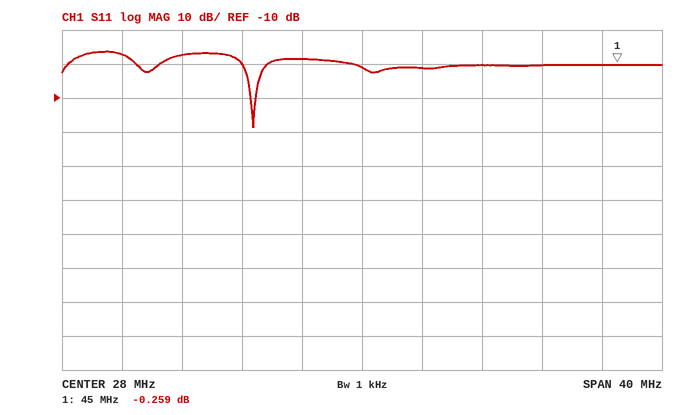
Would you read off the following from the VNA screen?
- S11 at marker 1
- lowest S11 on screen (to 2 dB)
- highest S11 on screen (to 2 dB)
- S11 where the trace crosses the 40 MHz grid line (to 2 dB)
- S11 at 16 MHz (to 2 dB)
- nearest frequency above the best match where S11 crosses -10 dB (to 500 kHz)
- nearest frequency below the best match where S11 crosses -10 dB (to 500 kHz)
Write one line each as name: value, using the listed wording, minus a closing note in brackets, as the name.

S11 at marker 1: -0.259 dB
lowest S11 on screen: -18 dB
highest S11 on screen: 4 dB
S11 where the trace crosses the 40 MHz grid line: 0 dB
S11 at 16 MHz: 2 dB
nearest frequency above the best match where S11 crosses -10 dB: 21.0 MHz
nearest frequency below the best match where S11 crosses -10 dB: 20.5 MHz
